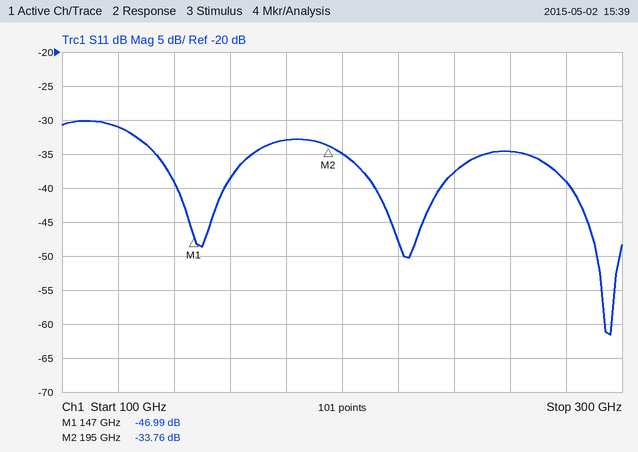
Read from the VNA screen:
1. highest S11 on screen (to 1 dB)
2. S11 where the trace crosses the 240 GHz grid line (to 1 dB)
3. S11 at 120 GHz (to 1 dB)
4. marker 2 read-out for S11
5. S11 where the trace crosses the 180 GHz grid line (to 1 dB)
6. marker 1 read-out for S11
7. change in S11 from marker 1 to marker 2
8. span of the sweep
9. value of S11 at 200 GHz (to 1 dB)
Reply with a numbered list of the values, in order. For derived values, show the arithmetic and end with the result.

1. -30 dB
2. -38 dB
3. -31 dB
4. -33.76 dB
5. -33 dB
6. -46.99 dB
7. -33.76 − (-46.99) = 13.23 dB
8. 200 GHz
9. -35 dB
